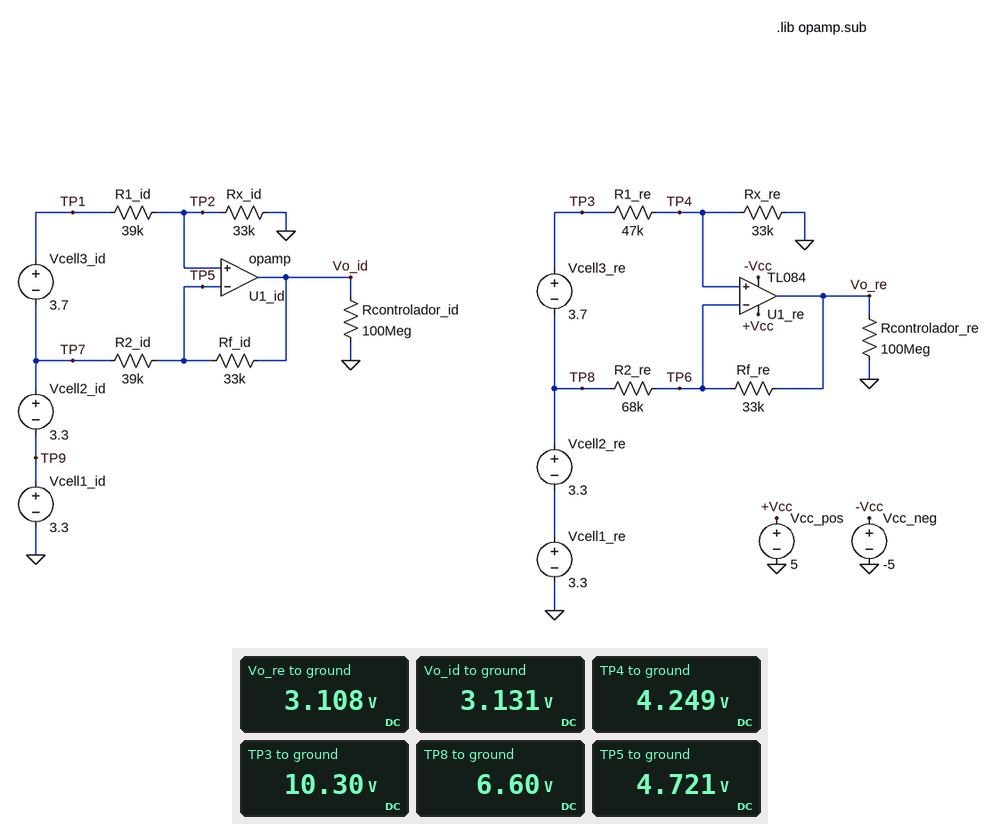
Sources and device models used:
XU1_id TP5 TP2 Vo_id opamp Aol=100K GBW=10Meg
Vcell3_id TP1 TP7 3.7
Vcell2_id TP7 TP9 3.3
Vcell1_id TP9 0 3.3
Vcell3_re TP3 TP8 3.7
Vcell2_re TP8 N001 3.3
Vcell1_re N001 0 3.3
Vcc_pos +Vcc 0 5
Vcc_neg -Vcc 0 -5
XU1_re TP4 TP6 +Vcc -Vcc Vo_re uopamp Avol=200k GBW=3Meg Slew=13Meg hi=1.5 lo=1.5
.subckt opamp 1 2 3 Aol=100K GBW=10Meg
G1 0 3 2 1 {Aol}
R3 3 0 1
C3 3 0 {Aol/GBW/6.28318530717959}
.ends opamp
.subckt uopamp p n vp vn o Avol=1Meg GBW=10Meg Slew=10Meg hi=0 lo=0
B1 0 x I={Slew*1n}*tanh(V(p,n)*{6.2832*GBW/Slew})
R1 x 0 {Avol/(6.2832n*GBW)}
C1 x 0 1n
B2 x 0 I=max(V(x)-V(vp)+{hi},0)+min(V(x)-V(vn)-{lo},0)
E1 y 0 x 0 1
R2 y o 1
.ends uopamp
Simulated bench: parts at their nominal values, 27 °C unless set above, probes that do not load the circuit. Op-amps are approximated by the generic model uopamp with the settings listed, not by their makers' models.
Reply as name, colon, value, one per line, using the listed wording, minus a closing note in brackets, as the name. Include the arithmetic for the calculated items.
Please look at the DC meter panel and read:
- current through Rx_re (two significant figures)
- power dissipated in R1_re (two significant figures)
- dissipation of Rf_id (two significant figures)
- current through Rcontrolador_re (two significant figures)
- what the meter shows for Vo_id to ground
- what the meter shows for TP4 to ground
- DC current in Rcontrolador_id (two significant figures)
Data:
current through Rx_re: (4.249 V) / 33 kΩ = 130 µA
power dissipated in R1_re: (10.3 V - 4.249 V)^2 / 47 kΩ = 780 µW
dissipation of Rf_id: (4.721 V - 3.131 V)^2 / 33 kΩ = 77 µW
current through Rcontrolador_re: (3.108 V) / 100 MΩ = 31 nA
what the meter shows for Vo_id to ground: 3.131 V
what the meter shows for TP4 to ground: 4.249 V
DC current in Rcontrolador_id: (3.131 V) / 100 MΩ = 31 nA
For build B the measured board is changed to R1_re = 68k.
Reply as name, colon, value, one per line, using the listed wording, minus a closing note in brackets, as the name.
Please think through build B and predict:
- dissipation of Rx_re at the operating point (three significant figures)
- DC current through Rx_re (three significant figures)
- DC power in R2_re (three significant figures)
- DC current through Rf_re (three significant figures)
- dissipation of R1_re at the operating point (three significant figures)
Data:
dissipation of Rx_re at the operating point: 343 µW
DC current through Rx_re: 102 µA
DC power in R2_re: 154 µW
DC current through Rf_re: 47.6 µA
dissipation of R1_re at the operating point: 707 µW
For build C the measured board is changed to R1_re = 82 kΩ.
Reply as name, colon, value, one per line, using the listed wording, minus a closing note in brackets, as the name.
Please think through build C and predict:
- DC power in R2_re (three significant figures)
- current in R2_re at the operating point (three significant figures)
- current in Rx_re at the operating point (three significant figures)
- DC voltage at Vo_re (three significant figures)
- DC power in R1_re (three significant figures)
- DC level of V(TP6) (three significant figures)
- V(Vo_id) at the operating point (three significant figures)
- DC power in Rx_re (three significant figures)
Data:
DC power in R2_re: 195 µW
current in R2_re at the operating point: 53.6 µA
current in Rx_re at the operating point: 89.6 µA
DC voltage at Vo_re: 1.19 V
DC power in R1_re: 658 µW
DC level of V(TP6): 2.96 V
V(Vo_id) at the operating point: 3.13 V
DC power in Rx_re: 265 µW
